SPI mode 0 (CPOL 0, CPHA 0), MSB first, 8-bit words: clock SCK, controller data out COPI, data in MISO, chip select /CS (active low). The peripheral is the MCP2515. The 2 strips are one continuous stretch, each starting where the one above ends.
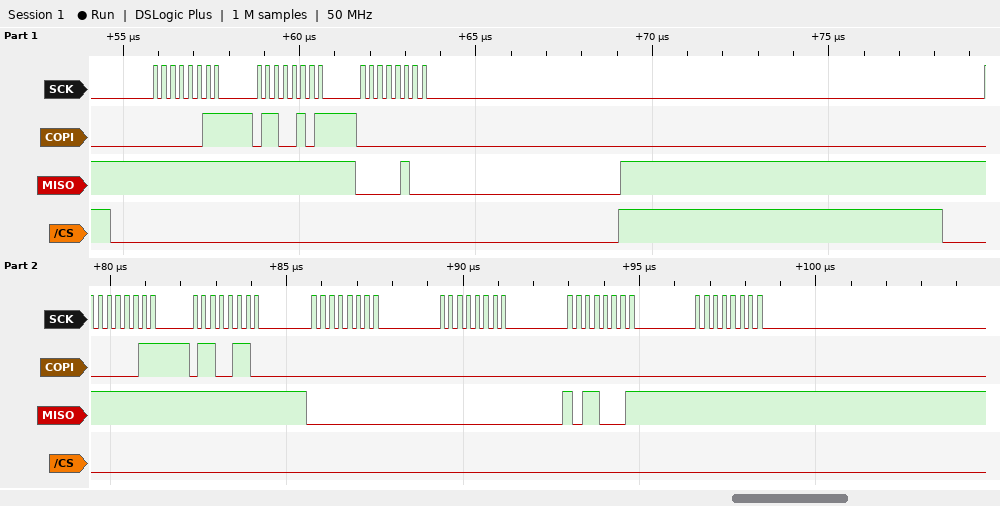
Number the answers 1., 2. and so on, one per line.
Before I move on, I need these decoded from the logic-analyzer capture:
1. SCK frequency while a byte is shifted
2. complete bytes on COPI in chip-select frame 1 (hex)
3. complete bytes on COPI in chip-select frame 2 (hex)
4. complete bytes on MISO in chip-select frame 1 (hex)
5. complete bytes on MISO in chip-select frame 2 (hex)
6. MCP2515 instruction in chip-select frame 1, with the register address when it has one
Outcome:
1. 4 MHz
2. 03 65 00
3. 03 66 00 00 00 00
4. FF FF 04
5. FF FF 00 00 B1 FF
6. READ 0x65
